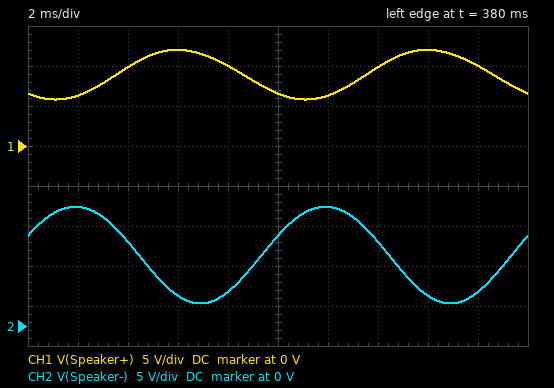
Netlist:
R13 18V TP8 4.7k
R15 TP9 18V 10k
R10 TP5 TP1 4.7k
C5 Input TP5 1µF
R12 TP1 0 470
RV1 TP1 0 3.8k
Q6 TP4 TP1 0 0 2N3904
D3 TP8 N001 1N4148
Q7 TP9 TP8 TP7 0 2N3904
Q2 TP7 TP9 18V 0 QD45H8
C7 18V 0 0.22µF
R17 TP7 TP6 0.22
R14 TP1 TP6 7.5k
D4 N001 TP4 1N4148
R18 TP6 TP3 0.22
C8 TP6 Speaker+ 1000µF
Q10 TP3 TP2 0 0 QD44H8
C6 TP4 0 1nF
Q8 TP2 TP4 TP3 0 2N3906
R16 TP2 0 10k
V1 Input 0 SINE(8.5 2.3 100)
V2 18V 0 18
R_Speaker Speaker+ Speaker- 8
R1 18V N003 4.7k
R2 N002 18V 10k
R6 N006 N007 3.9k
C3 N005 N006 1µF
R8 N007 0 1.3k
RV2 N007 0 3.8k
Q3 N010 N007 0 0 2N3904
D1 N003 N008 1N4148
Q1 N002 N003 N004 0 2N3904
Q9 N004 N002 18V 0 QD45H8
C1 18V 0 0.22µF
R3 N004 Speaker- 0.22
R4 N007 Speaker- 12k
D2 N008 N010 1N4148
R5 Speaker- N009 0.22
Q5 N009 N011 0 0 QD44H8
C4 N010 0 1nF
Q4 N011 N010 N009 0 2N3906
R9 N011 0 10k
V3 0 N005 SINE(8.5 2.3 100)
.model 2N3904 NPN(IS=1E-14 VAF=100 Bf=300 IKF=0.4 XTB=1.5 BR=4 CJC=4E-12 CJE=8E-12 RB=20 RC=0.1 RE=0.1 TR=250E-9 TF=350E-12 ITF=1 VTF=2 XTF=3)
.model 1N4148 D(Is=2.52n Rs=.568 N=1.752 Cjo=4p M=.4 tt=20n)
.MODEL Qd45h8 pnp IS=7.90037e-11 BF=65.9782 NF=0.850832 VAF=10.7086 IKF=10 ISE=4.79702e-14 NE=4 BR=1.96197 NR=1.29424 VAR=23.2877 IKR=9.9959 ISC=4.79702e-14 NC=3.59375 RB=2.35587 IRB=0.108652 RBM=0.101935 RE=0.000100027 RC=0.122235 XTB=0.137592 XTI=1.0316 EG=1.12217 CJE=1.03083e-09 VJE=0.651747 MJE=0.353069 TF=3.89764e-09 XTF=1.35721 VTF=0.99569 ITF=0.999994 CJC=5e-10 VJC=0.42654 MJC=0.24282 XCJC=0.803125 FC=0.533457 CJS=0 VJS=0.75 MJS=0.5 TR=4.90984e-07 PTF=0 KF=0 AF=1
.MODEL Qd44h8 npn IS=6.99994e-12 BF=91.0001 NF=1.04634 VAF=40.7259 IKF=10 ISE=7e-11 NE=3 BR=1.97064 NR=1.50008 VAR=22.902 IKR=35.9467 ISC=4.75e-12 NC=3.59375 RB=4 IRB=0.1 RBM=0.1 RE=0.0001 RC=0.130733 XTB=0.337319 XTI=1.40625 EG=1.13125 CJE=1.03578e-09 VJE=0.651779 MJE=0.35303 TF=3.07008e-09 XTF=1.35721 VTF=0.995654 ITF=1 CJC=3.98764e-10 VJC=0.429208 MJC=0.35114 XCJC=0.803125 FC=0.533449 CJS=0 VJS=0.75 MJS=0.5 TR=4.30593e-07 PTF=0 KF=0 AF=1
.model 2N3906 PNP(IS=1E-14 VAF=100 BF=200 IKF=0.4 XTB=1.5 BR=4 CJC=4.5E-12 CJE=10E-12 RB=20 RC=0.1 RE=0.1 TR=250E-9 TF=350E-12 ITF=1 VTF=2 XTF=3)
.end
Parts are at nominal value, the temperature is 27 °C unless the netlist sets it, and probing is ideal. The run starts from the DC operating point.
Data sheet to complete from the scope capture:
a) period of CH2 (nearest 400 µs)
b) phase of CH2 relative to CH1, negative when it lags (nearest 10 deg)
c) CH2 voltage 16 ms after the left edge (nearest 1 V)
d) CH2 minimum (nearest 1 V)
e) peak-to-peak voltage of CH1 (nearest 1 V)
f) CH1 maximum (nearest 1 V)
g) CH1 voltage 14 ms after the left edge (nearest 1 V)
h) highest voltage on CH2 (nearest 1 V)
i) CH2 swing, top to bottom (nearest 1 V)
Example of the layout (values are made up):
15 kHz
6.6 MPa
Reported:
10.0 ms
150 deg
4 V
3 V
6 V
12 V
10 V
15 V
12 V
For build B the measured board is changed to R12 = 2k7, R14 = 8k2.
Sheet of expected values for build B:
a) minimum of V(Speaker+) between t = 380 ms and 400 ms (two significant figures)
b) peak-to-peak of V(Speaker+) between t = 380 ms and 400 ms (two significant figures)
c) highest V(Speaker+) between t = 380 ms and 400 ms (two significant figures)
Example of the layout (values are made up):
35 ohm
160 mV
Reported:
5.2 V
7.5 V
13 V
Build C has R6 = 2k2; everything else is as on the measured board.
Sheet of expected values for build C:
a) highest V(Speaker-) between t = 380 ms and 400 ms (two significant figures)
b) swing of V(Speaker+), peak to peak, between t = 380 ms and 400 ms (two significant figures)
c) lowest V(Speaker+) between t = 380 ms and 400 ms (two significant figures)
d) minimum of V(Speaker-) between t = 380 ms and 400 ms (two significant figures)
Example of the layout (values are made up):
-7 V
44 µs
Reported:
17 V
5.8 V
6.0 V
1.1 V
